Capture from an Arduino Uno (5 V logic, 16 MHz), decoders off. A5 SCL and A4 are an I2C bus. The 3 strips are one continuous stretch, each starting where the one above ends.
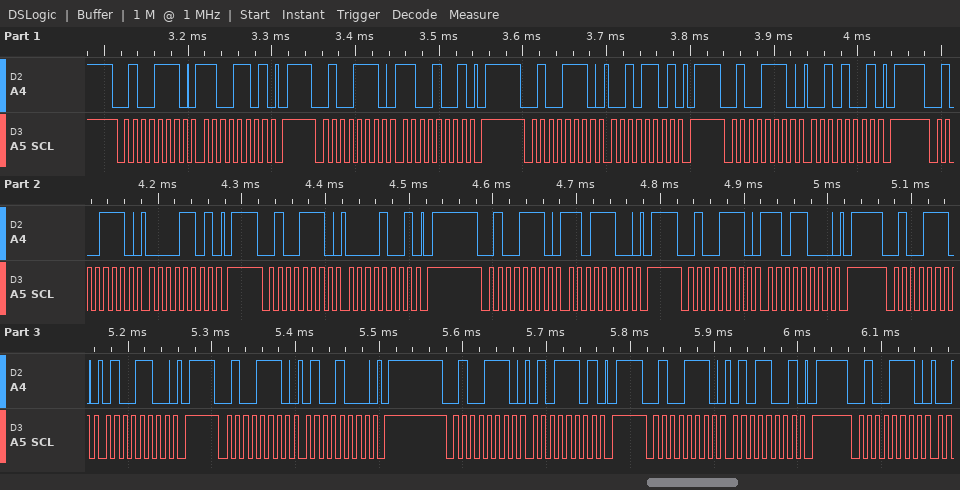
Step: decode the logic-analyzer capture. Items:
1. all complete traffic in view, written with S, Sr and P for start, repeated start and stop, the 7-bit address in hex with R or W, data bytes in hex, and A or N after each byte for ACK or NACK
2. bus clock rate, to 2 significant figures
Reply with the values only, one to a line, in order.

S 27W A CD A P S 27W A C9 A P S 27W A 2D A P S 27W A 29 A P S 27W A 0D A P S 27W A 09 A P S 27W A DC A P S 27W A D8 A P S 27W A 4C A P S 27W A 48 A P S 27W A 5D A P S 27W A 59 A P S 27W A
100 kHz
